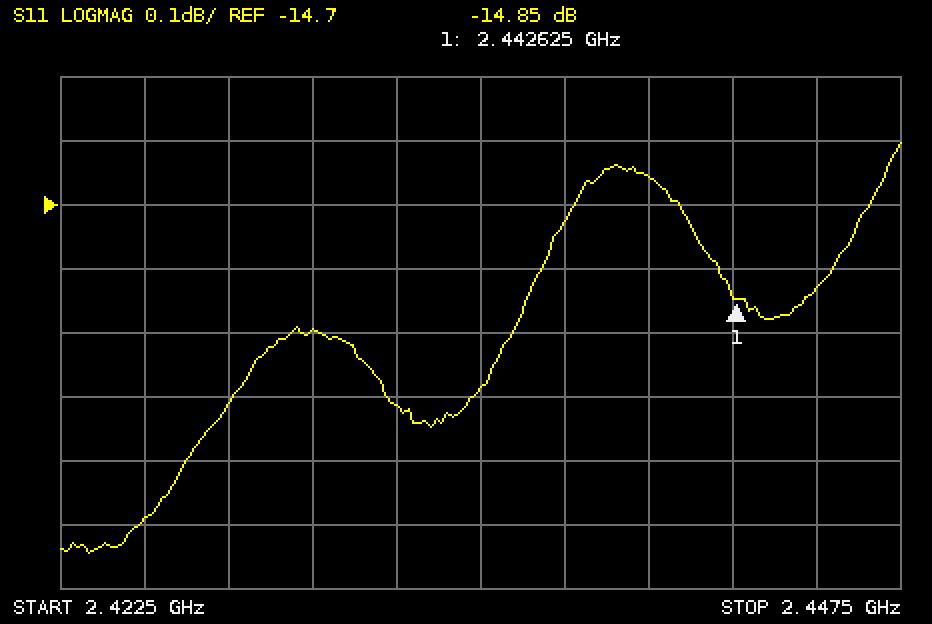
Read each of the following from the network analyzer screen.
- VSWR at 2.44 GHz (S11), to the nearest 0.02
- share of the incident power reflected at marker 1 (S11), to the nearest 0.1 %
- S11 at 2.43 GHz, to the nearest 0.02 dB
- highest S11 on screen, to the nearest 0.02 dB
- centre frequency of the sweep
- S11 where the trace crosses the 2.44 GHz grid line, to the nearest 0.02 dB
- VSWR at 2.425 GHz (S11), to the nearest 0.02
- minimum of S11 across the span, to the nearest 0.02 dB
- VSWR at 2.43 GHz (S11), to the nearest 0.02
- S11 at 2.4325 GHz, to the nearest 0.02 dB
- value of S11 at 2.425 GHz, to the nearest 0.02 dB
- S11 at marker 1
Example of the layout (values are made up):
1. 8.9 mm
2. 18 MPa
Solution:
1. 1.46
2. 3.3 %
3. -14.90 dB
4. -14.60 dB
5. 2.435 GHz
6. -14.66 dB
7. 1.42
8. -15.24 dB
9. 1.44
10. -15.02 dB
11. -15.18 dB
12. -14.85 dB
